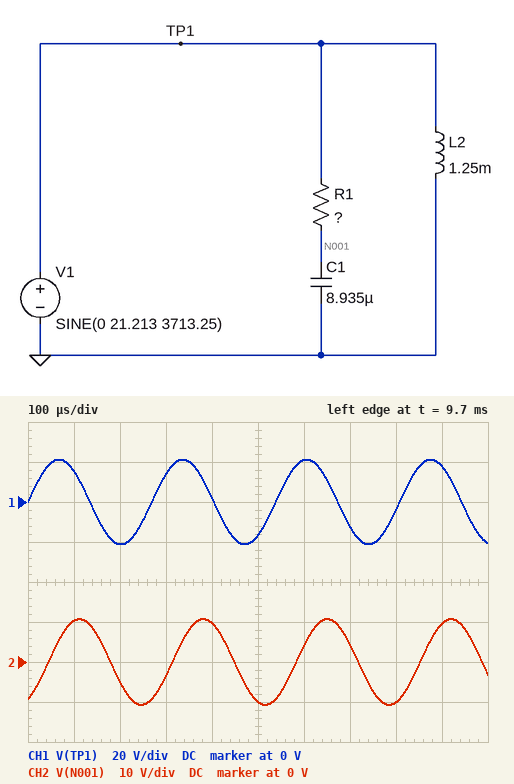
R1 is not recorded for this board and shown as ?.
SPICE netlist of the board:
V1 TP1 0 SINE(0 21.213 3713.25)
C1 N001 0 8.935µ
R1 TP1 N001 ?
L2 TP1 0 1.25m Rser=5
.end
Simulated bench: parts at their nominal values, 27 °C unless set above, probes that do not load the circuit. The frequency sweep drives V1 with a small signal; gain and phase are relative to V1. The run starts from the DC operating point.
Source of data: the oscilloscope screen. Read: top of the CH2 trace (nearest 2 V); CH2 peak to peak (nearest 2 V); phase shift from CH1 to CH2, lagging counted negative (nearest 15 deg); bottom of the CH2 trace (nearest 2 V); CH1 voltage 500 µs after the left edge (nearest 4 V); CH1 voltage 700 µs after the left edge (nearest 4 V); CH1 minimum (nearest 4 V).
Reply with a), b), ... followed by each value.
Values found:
a) 10 V
b) 22 V
c) -60 deg
d) -10 V
e) -16 V
f) -12 V
g) -20 V
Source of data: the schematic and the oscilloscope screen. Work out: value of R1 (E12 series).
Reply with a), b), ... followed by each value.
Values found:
a) 8.2 Ω
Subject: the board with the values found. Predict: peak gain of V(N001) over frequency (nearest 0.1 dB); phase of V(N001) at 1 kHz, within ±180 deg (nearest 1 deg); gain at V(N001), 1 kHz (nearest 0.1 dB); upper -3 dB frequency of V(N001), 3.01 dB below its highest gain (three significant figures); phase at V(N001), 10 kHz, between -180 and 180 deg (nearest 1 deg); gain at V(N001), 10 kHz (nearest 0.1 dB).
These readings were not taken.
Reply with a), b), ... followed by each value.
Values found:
a) 0 dB
b) -25 deg
c) -0.8 dB
d) 2.17 kHz
e) -78 deg
f) -13.5 dB
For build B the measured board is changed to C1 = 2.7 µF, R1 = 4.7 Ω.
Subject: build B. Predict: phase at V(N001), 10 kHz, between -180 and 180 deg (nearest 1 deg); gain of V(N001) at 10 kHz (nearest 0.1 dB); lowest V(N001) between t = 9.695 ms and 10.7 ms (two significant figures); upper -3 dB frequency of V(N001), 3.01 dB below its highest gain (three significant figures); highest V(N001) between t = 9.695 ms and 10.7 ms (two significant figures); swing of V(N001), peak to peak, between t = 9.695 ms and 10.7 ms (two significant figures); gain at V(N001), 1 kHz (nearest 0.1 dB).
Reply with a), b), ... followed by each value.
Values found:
a) -39 deg
b) -2.1 dB
c) -20 V
d) 12.5 kHz
e) 20 V
f) 41 V
g) 0 dB
